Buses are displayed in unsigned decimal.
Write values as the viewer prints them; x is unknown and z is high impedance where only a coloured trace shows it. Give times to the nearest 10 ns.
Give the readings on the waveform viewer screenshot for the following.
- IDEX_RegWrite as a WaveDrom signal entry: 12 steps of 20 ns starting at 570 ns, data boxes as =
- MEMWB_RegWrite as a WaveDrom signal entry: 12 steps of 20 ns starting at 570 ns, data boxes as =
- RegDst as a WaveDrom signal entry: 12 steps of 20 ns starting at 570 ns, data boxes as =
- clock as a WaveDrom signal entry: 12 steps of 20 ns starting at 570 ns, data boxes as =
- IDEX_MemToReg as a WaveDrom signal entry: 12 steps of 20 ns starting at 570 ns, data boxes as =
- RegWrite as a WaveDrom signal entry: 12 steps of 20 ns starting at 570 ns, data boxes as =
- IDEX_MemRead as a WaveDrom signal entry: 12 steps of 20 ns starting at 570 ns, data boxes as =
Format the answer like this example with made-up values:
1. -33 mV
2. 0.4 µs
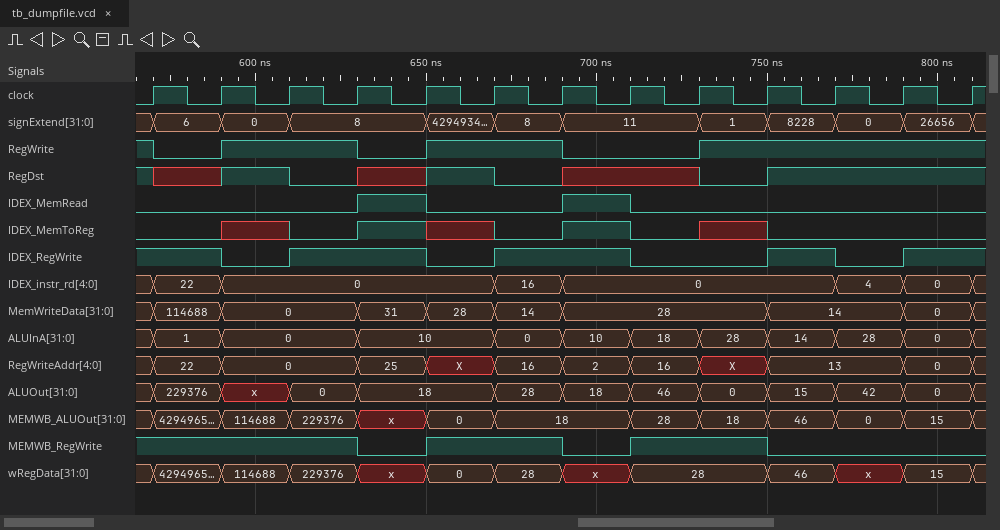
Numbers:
1. {name: 'IDEX_RegWrite', wave: '101.01.0.101'}
2. {name: 'MEMWB_RegWrite', wave: '1..01.01.0..'}
3. {name: 'RegDst', wave: 'x10x10x.01..'}
4. {name: 'clock', wave: 'p...........'}
5. {name: 'IDEX_MemToReg', wave: '0x01x010x0..'}
6. {name: 'RegWrite', wave: '01.01.0.1...'}
7. {name: 'IDEX_MemRead', wave: '0..10.10....'}
